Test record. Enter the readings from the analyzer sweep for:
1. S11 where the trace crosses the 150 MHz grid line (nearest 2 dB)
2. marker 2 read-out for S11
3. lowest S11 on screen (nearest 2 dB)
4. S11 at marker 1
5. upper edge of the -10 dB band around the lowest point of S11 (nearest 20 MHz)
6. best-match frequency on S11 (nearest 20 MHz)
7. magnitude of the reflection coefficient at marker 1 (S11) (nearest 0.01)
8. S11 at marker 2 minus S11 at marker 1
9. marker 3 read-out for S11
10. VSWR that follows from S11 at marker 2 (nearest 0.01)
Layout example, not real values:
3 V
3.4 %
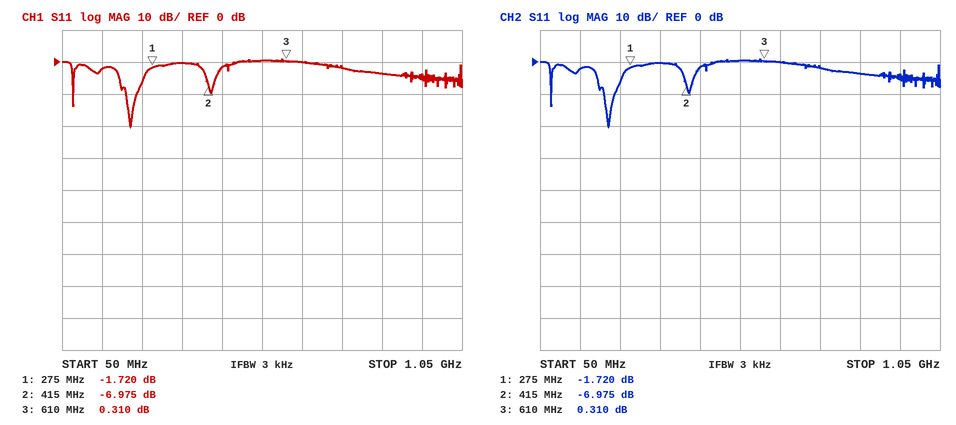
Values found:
-2 dB
-6.975 dB
-20 dB
-1.720 dB
240 MHz
220 MHz
0.82
-5.255 dB
0.310 dB
2.62
